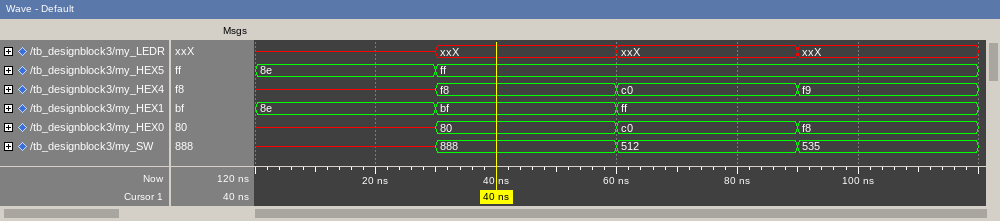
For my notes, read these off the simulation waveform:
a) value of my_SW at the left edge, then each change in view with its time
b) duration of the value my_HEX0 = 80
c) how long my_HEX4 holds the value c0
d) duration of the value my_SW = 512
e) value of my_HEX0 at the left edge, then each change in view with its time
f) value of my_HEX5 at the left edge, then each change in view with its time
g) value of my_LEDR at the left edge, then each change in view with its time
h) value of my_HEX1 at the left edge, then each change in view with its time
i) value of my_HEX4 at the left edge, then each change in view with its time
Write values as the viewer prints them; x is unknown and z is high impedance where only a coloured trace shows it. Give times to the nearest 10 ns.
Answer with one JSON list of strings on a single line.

["x, 888 at 30 ns, 512 at 60 ns, 535 at 90 ns", "30 ns", "30 ns", "30 ns", "x, 80 at 30 ns, c0 at 60 ns, f8 at 90 ns", "8e, ff at 30 ns", "x, xxX at 30 ns, xxX at 60 ns, xxX at 90 ns", "8e, bf at 30 ns, ff at 60 ns", "x, f8 at 30 ns, c0 at 60 ns, f9 at 90 ns"]
